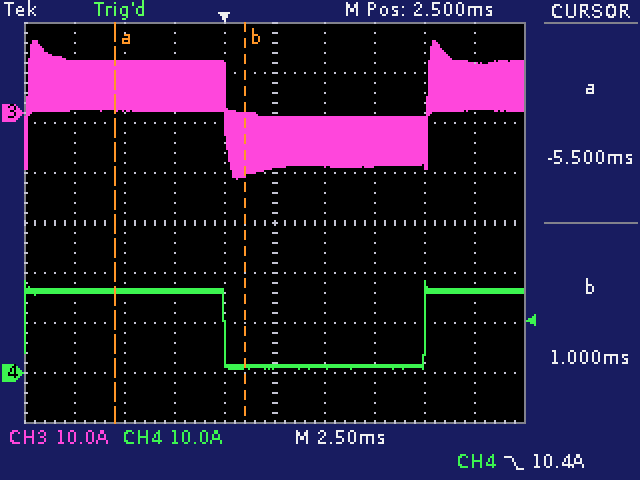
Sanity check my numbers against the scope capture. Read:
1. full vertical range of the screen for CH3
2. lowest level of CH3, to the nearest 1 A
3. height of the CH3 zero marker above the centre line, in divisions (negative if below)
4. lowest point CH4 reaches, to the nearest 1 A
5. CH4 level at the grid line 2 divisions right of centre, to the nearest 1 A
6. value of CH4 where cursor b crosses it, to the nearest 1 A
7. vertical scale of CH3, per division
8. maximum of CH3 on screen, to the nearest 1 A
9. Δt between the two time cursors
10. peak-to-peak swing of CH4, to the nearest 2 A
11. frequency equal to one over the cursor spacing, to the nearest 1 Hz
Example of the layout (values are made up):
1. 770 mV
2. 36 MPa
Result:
1. 80 A
2. -13 A
3. +2.2 div
4. 1 A
5. 1 A
6. 1 A
7. 10 A
8. 14 A
9. 6.50 ms
10. 18 A
11. 154 Hz
